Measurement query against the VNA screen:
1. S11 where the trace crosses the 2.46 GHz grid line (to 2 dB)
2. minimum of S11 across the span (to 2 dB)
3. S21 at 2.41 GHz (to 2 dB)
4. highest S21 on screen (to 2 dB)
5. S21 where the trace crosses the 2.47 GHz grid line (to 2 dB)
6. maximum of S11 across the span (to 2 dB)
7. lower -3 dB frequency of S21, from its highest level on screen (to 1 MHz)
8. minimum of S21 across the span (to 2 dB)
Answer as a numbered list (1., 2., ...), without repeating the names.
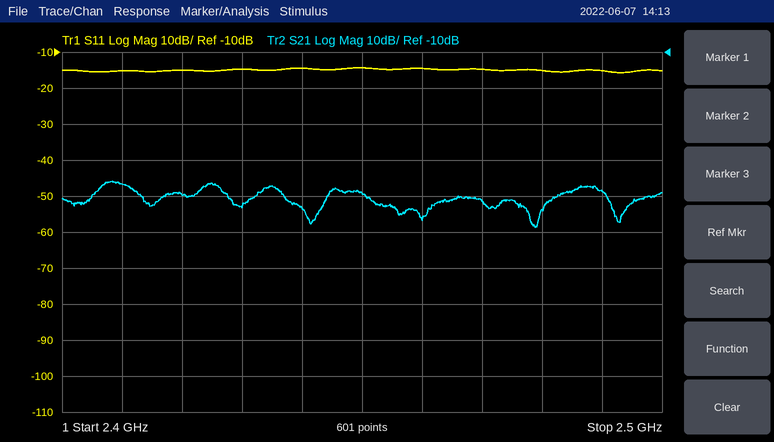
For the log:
1. -14 dB
2. -16 dB
3. -46 dB
4. -46 dB
5. -52 dB
6. -14 dB
7. 2.406 GHz
8. -58 dB
